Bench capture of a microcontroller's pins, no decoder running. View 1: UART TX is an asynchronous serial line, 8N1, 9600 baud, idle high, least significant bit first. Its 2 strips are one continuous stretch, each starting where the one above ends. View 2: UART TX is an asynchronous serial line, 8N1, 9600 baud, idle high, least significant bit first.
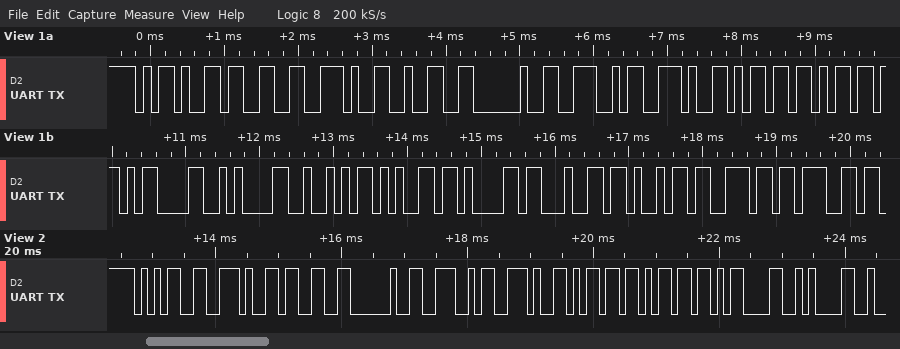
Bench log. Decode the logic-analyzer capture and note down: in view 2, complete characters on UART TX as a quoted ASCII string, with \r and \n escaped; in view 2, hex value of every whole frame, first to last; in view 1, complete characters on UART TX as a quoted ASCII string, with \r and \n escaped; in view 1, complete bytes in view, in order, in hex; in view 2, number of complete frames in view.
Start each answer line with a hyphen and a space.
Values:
- "5.3 N.mm\r\n"
- 0x35 0x2E 0x33 0x20 0x4E 0x2E 0x6D 0x6D 0x0D 0x0A
- "-3.2 N.mm\r\nReading"
- 2D 33 2E 32 20 4E 2E 6D 6D 0D 0A 52 65 61 64 69 6E 67
- 10
